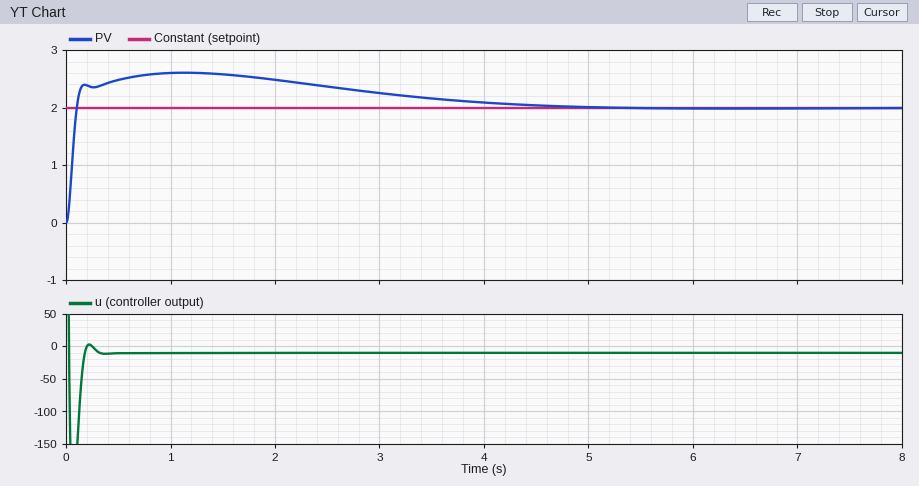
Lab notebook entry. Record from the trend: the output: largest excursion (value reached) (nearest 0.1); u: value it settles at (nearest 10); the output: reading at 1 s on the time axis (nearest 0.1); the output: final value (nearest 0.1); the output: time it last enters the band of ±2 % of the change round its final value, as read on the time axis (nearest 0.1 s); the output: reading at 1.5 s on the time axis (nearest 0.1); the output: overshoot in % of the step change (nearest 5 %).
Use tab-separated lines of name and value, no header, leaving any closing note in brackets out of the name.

the output: largest excursion (value reached)	2.6
u: value it settles at	-10
the output: reading at 1 s on the time axis	2.6
the output: final value	2.0
the output: time it last enters the band of ±2 % of the change round its final value, as read on the time axis	4.5 s
the output: reading at 1.5 s on the time axis	2.6
the output: overshoot in % of the step change	30 %
